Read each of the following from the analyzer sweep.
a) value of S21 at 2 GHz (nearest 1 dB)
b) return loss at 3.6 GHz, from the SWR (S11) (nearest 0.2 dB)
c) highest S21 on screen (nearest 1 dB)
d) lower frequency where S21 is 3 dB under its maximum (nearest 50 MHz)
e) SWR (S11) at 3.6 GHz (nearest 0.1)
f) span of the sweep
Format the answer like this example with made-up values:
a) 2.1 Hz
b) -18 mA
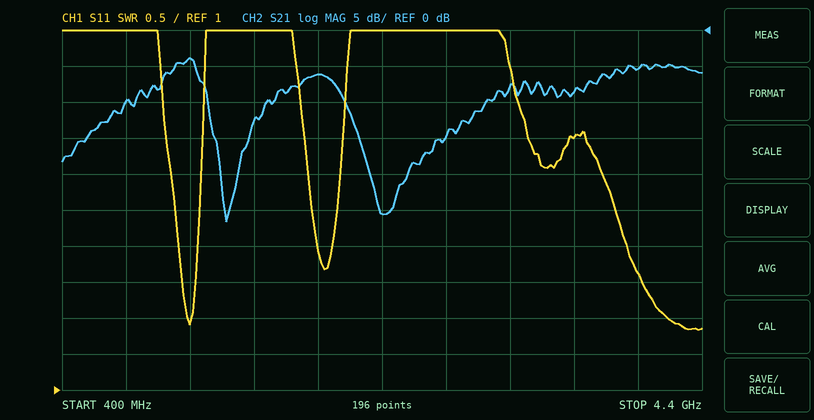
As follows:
a) -6 dB
b) 4.0 dB
c) -4 dB
d) 1.05 GHz
e) 4.5
f) 4 GHz
